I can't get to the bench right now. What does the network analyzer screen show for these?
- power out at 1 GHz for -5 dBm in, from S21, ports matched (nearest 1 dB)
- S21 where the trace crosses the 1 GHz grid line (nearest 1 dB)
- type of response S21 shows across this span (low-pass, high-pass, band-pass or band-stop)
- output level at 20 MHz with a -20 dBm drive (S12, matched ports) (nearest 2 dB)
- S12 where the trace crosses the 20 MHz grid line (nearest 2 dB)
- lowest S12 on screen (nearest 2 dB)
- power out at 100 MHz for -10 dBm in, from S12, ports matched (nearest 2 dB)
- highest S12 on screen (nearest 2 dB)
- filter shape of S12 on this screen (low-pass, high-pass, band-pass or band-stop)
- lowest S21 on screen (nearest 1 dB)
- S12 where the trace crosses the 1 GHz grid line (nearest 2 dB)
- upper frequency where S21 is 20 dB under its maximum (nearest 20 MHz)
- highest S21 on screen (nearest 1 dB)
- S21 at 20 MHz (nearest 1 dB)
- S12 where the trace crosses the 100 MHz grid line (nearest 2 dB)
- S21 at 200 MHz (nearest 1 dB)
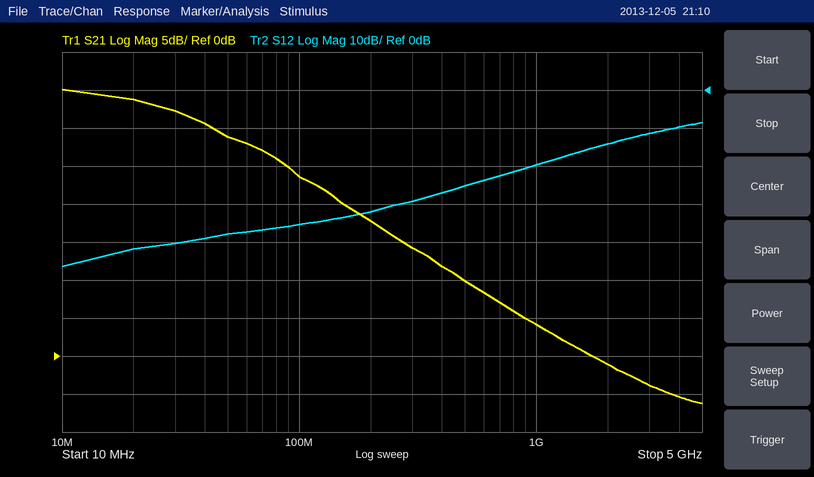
-1 dBm
4 dB
low-pass
-62 dBm
-42 dB
-46 dB
-46 dBm
-8 dB
high-pass
-6 dB
-20 dB
280 MHz
35 dB
34 dB
-36 dB
18 dB
